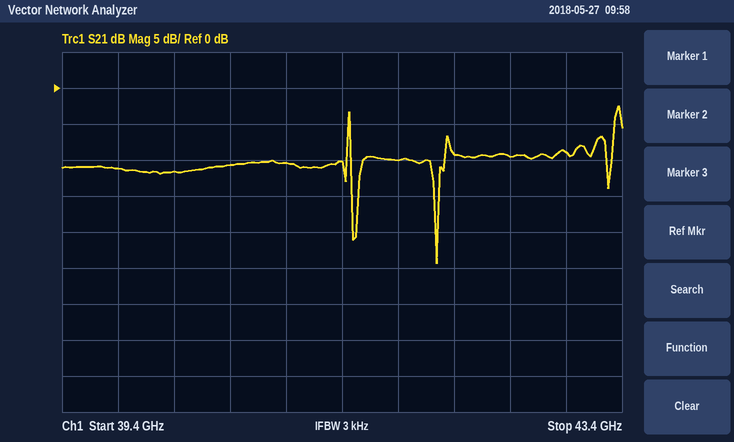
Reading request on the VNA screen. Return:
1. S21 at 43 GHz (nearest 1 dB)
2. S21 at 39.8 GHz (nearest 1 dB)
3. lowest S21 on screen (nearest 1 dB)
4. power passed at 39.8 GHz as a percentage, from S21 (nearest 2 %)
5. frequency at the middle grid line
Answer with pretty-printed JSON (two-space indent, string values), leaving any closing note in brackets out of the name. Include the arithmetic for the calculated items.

{
  "S21 at 43 GHz": "-9 dB",
  "S21 at 39.8 GHz": "-11 dB",
  "lowest S21 on screen": "-24 dB",
  "power passed at 39.8 GHz as a percentage, from S21": "10^(-11/10) ≈ 8 %",
  "frequency at the middle grid line": "41.4 GHz"
}
